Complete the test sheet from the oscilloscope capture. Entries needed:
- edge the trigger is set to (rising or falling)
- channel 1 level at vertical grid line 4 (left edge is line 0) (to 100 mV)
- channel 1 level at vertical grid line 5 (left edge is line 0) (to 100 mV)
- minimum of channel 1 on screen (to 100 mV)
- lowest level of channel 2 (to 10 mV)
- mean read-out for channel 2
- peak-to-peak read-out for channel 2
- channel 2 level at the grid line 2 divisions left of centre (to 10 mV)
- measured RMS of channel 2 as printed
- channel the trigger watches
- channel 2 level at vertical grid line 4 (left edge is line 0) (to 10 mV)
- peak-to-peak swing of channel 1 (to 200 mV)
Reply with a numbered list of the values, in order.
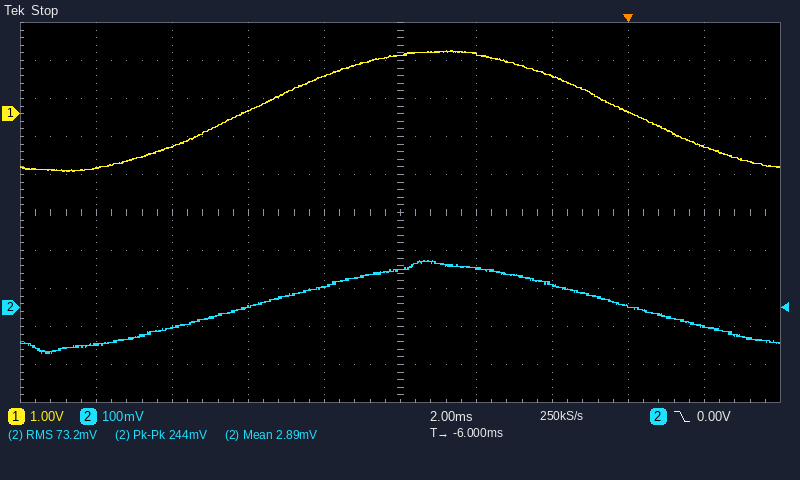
1. falling
2. 1.0 V
3. 1.5 V
4. -1.5 V
5. -120 mV
6. 2.89 mV
7. 244 mV
8. 0 mV
9. 73.2 mV
10. channel 2
11. 60 mV
12. 3.2 V
